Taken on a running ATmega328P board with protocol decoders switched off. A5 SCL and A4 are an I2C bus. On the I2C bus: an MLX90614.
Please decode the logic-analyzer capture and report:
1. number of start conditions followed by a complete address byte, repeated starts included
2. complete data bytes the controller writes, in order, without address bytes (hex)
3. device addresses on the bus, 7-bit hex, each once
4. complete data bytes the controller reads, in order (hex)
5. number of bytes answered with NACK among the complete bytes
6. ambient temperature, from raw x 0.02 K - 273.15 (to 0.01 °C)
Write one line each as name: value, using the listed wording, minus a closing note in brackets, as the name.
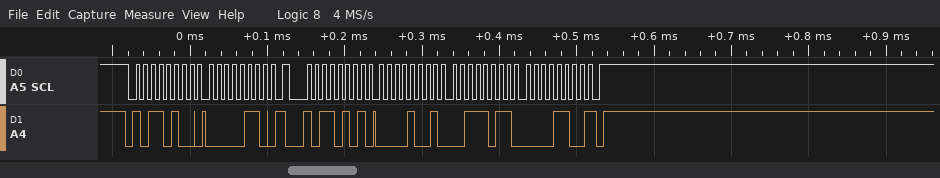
number of start conditions followed by a complete address byte, repeated starts included: 2
complete data bytes the controller writes, in order, without address bytes: 06
device addresses on the bus, 7-bit hex, each once: 0x5A
complete data bytes the controller reads, in order: 09 3B 0C
number of bytes answered with NACK among the complete bytes: 1
ambient temperature, from raw x 0.02 K - 273.15: 29.11 °C
